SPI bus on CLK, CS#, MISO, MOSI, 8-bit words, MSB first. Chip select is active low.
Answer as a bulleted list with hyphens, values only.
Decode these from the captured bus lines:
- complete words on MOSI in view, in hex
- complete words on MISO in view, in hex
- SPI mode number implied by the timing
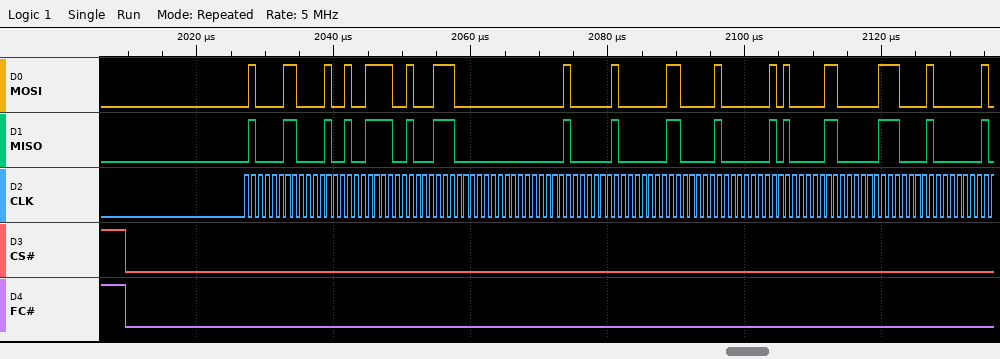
- 43, 09, 3C, 8E, 00, 01, 02, 03, 04, 05, 06, 07, 08
- 43, 09, 3C, 8E, 00, 01, 02, 03, 04, 05, 06, 07, 08
- 0
